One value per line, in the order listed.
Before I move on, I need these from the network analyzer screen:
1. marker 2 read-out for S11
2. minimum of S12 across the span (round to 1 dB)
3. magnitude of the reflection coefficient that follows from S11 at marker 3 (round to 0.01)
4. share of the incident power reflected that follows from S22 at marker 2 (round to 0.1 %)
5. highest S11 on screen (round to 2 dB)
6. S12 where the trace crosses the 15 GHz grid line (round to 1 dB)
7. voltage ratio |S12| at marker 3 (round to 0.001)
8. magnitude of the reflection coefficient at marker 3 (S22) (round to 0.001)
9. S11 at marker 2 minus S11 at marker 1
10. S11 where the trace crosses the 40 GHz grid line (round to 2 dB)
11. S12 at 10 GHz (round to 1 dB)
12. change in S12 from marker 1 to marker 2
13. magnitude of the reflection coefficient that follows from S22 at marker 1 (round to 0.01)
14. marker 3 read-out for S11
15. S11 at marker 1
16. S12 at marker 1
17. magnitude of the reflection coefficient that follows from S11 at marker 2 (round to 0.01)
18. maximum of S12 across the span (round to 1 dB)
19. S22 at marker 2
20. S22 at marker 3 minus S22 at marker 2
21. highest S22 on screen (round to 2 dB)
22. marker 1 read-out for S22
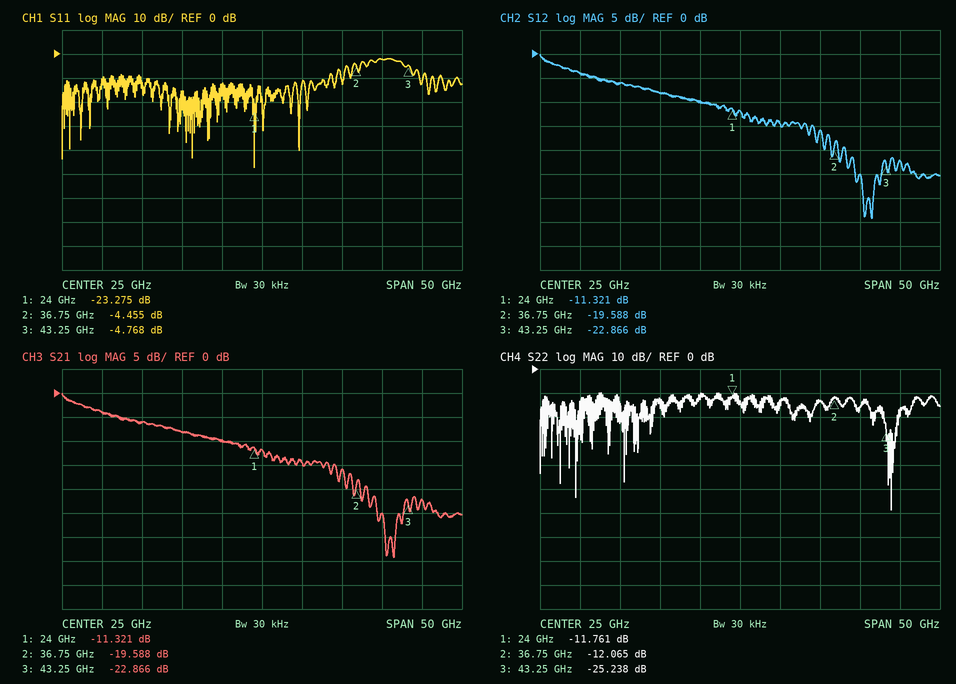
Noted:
-4.455 dB
-34 dB
0.58
6.2 %
-2 dB
-8 dB
0.072
0.055
18.820 dB
-2 dB
-6 dB
-8.267 dB
0.26
-4.768 dB
-23.275 dB
-11.321 dB
0.60
0 dB
-12.065 dB
-13.173 dB
-10 dB
-11.761 dB
